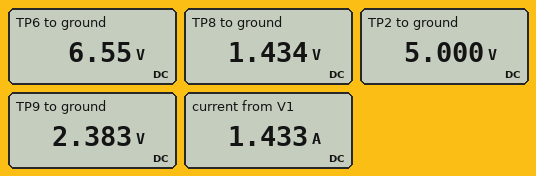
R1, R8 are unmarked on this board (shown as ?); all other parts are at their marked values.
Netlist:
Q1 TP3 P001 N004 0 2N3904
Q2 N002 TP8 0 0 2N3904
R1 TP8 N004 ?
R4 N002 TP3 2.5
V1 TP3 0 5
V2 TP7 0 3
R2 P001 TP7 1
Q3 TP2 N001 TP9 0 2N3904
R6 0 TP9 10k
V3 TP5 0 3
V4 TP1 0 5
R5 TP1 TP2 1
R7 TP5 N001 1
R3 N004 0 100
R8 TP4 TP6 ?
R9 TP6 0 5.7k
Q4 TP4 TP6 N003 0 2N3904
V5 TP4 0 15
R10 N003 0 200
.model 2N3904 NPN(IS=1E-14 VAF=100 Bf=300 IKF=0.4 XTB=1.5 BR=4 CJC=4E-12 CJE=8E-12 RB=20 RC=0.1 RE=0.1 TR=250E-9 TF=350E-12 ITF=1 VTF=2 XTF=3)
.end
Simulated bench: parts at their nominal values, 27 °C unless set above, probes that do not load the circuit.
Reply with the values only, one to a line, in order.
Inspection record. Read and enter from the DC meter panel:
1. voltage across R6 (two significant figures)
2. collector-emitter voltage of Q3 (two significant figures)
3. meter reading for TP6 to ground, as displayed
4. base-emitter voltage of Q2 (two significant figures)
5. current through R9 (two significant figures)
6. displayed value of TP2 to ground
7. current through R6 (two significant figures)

2.4 V
2.6 V
6.55 V
1.4 V
1.1 mA
5.000 V
240 µA
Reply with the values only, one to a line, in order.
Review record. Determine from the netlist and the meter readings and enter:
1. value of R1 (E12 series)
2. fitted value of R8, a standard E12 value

39 Ω
6.8 kΩ
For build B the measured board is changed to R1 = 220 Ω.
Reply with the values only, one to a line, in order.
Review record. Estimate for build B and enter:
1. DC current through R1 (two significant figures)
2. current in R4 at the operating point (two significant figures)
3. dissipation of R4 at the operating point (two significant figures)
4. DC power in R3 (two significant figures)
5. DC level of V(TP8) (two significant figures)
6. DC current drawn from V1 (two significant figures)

5.6 mA
660 mA
1.1 W
51 mW
1.0 V
690 mA
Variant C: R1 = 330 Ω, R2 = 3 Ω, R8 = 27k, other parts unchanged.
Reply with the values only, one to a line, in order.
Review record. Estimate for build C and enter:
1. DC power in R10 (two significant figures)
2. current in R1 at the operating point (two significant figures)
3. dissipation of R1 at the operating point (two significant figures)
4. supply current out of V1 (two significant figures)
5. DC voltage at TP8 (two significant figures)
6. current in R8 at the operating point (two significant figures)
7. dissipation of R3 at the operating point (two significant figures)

16 mW
3.9 mA
5.0 mW
550 mA
970 mV
460 µA
51 mW
